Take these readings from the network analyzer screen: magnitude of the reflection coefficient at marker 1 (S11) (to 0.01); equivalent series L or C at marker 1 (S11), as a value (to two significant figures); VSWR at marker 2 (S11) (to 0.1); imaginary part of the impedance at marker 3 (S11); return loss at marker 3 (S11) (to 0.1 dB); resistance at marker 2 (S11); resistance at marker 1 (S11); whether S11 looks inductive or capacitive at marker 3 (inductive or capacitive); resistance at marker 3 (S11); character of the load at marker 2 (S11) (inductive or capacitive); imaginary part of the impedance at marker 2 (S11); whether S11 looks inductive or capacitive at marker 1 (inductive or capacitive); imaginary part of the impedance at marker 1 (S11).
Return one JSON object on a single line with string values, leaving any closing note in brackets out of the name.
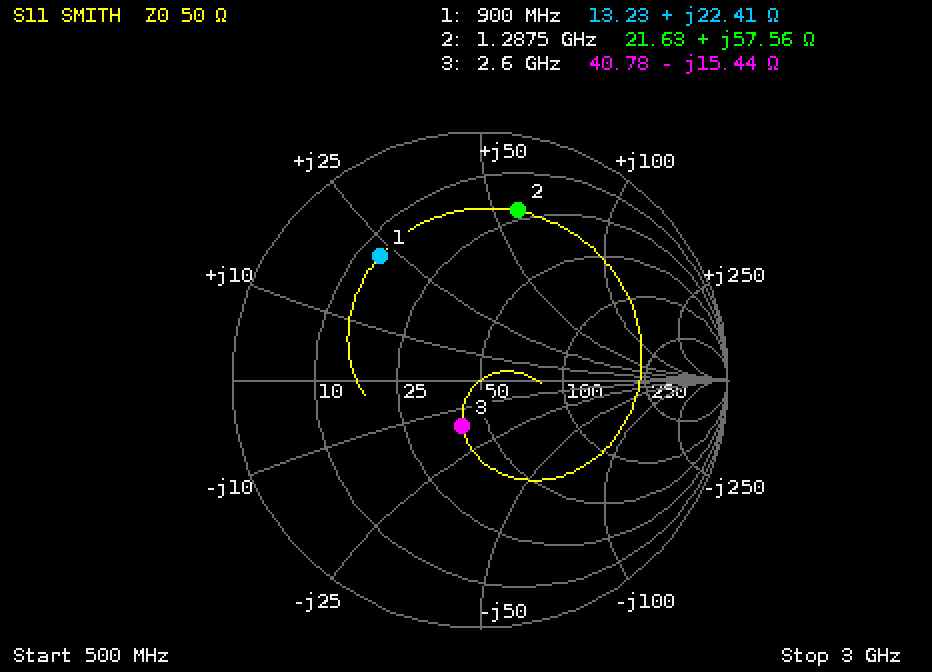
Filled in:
{"magnitude of the reflection coefficient at marker 1 (S11)": "0.64", "equivalent series L or C at marker 1 (S11), as a value": "4.0 nH", "VSWR at marker 2 (S11)": "5.6", "imaginary part of the impedance at marker 3": "-15.44 Ω", "return loss at marker 3 (S11)": "14.2 dB", "resistance at marker 2": "21.63 Ω", "resistance at marker 1": "13.23 Ω", "whether S11 looks inductive or capacitive at marker 3": "capacitive", "resistance at marker 3": "40.78 Ω", "character of the load at marker 2 (S11)": "inductive", "imaginary part of the impedance at marker 2": "+57.56 Ω", "whether S11 looks inductive or capacitive at marker 1": "inductive", "imaginary part of the impedance at marker 1": "+22.41 Ω"}
